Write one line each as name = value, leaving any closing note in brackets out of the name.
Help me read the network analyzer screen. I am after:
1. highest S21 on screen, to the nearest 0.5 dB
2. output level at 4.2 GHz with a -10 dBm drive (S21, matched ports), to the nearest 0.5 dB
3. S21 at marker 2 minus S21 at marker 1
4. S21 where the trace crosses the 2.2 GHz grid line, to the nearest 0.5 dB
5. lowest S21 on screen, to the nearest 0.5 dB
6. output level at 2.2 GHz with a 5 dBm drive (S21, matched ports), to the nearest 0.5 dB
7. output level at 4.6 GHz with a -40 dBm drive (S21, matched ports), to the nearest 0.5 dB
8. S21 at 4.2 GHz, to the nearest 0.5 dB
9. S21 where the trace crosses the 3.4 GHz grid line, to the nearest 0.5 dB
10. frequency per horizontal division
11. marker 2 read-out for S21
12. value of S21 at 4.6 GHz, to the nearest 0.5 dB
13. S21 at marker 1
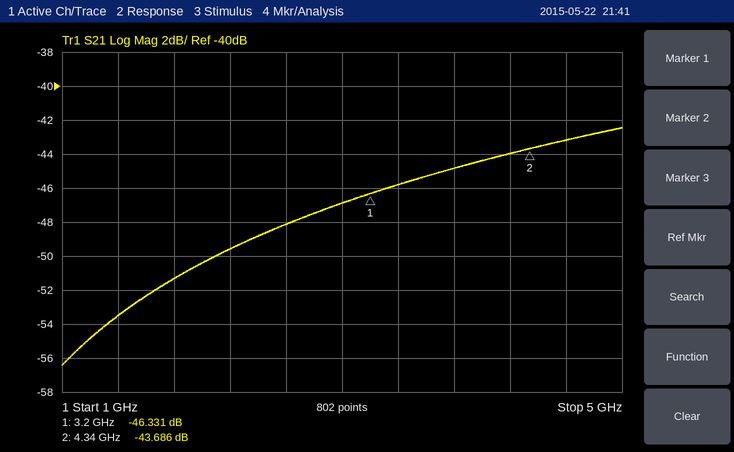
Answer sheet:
highest S21 on screen, to the nearest 0.5 dB = -42.5 dB
output level at 4.2 GHz with a -10 dBm drive (S21, matched ports), to the nearest 0.5 dB = -54.0 dBm
S21 at marker 2 minus S21 at marker 1 = 2.645 dB
S21 where the trace crosses the 2.2 GHz grid line, to the nearest 0.5 dB = -49.5 dB
lowest S21 on screen, to the nearest 0.5 dB = -56.5 dB
output level at 2.2 GHz with a 5 dBm drive (S21, matched ports), to the nearest 0.5 dB = -44.5 dBm
output level at 4.6 GHz with a -40 dBm drive (S21, matched ports), to the nearest 0.5 dB = -83.0 dBm
S21 at 4.2 GHz, to the nearest 0.5 dB = -44.0 dB
S21 where the trace crosses the 3.4 GHz grid line, to the nearest 0.5 dB = -46.0 dB
frequency per horizontal division = 400 MHz
marker 2 read-out for S21 = -43.686 dB
value of S21 at 4.6 GHz, to the nearest 0.5 dB = -43.0 dB
S21 at marker 1 = -46.331 dB
